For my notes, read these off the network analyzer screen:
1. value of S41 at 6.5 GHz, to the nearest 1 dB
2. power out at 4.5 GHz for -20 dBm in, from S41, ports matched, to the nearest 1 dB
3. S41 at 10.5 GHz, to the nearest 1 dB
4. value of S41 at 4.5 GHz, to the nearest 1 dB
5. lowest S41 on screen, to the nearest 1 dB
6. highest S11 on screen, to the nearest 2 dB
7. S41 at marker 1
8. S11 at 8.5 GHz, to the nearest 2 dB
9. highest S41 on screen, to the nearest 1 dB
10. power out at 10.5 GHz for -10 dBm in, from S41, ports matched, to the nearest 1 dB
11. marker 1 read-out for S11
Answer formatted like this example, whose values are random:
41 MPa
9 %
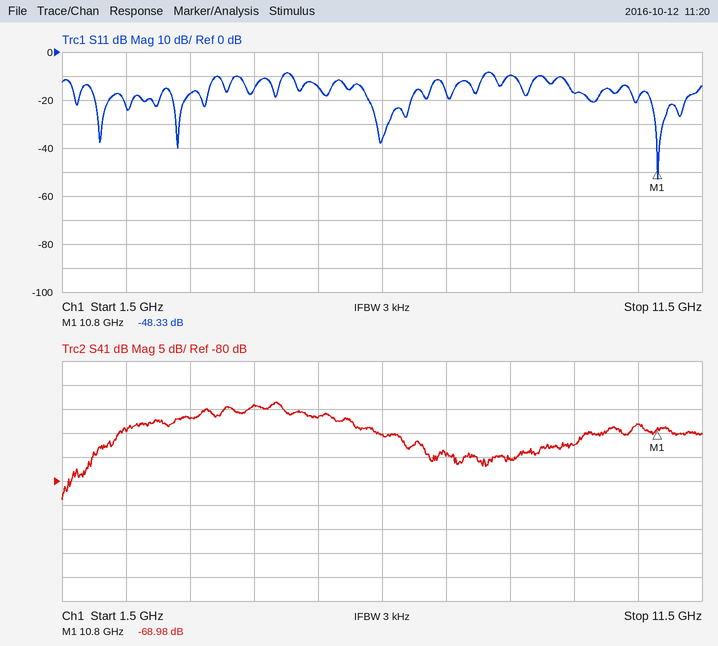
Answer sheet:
-70 dB
-84 dBm
-68 dB
-64 dB
-84 dB
-8 dB
-68.98 dB
-10 dB
-64 dB
-78 dBm
-48.33 dB
